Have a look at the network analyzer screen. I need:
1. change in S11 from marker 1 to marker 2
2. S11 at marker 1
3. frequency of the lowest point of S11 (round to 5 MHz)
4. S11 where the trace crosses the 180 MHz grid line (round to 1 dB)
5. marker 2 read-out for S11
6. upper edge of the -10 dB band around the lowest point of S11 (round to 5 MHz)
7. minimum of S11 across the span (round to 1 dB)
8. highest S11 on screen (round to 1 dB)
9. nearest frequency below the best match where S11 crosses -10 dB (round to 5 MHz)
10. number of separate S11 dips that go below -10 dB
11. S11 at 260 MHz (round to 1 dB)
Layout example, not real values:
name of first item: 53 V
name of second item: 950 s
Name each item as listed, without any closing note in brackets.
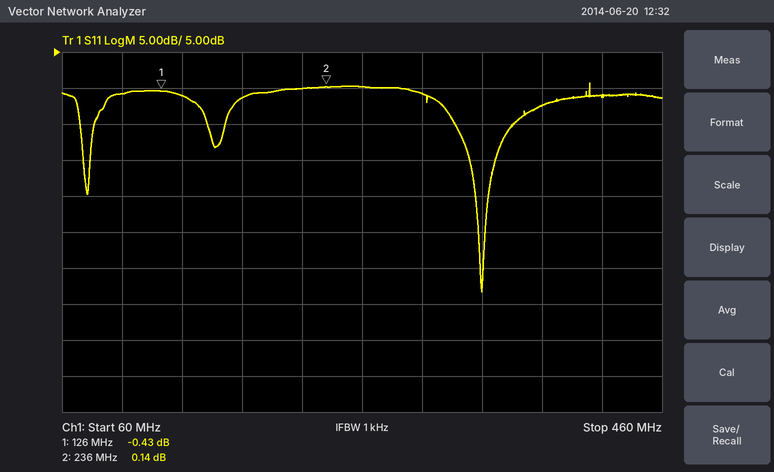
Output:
change in S11 from marker 1 to marker 2: 0.57 dB
S11 at marker 1: -0.43 dB
frequency of the lowest point of S11: 340 MHz
S11 where the trace crosses the 180 MHz grid line: -1 dB
marker 2 read-out for S11: 0.14 dB
upper edge of the -10 dB band around the lowest point of S11: 350 MHz
minimum of S11 across the span: -28 dB
highest S11 on screen: 1 dB
nearest frequency below the best match where S11 crosses -10 dB: 330 MHz
number of separate S11 dips that go below -10 dB: 2
S11 at 260 MHz: 0 dB
